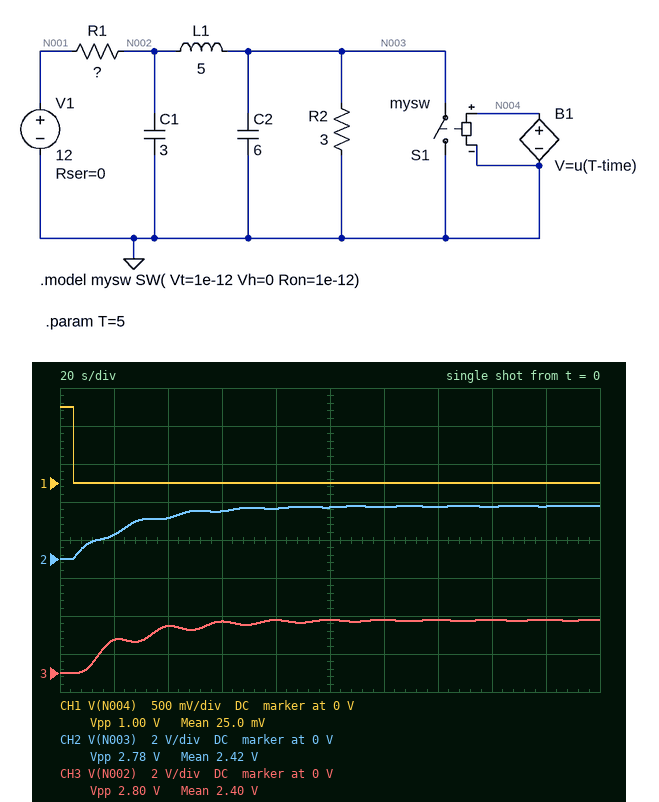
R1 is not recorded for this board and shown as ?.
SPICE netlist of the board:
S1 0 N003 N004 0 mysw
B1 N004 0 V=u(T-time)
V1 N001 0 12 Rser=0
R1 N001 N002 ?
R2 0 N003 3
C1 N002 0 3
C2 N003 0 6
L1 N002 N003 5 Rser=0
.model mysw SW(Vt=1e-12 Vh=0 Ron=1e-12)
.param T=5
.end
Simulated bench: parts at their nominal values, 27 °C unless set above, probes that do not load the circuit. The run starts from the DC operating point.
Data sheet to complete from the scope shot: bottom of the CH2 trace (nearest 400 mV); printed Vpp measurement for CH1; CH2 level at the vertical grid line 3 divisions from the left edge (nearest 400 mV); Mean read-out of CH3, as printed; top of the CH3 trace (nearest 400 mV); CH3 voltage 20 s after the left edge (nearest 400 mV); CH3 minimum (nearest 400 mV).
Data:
0 V
1.00 V
2.4 V
2.40 V
2.8 V
1.6 V
0 V
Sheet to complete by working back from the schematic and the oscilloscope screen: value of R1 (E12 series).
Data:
10 Ω
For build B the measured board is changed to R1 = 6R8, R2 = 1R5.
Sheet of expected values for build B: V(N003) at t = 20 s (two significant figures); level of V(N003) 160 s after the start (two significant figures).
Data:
1.4 V
2.2 V
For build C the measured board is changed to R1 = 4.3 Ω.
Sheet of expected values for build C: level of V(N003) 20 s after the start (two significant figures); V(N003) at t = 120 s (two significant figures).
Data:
2.7 V
4.9 V
